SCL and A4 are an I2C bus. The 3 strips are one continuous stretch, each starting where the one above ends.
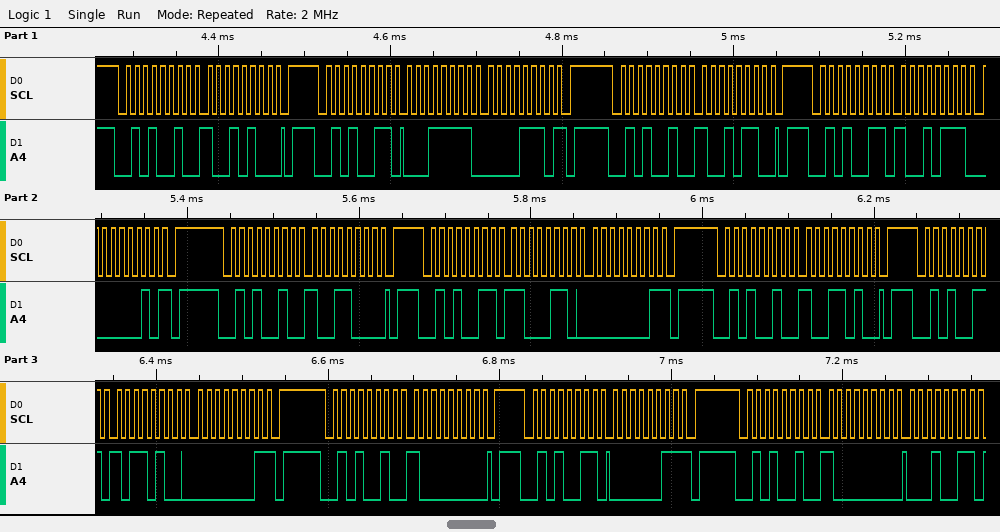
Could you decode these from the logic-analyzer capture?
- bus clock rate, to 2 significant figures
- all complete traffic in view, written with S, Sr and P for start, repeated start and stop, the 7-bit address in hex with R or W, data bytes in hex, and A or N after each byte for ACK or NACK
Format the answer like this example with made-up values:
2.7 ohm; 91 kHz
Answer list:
100 kHz; S 29W A 94 A P S 29R A 1F A 0E N P S 29W A 96 A P S 29R A 97 A 02 N P S 29W A 98 A P S 29R A C6 A 01 N P S 29W A 9A A P S 29R A B4 A 01 N P S 29W A 80 A P S 29R A 03 N P S 29W A 80 A 13 A
